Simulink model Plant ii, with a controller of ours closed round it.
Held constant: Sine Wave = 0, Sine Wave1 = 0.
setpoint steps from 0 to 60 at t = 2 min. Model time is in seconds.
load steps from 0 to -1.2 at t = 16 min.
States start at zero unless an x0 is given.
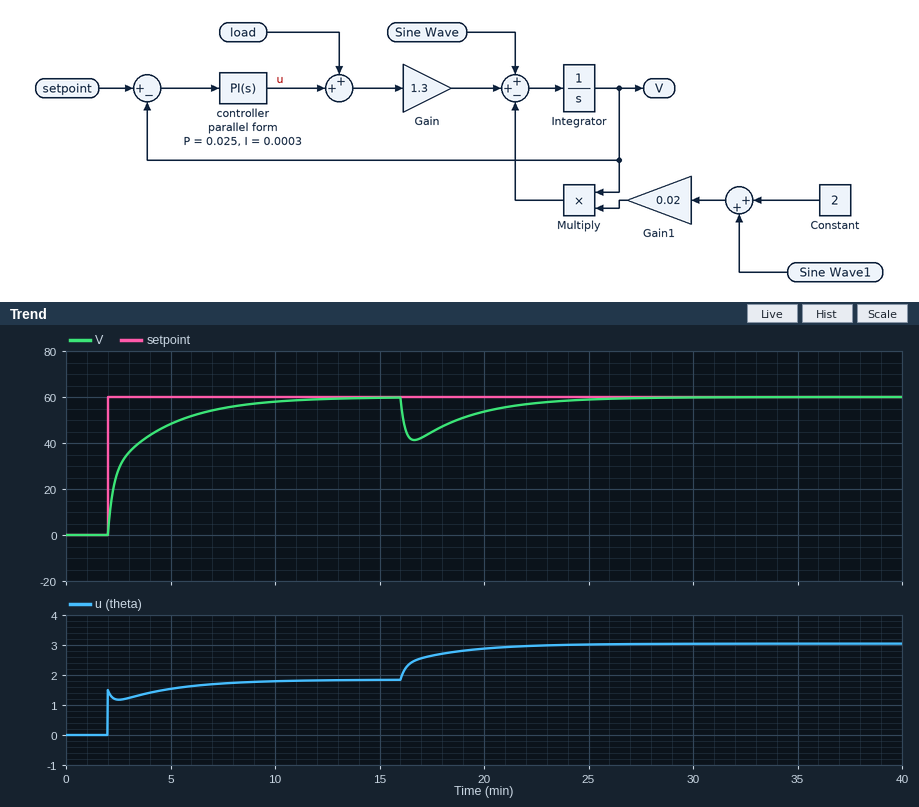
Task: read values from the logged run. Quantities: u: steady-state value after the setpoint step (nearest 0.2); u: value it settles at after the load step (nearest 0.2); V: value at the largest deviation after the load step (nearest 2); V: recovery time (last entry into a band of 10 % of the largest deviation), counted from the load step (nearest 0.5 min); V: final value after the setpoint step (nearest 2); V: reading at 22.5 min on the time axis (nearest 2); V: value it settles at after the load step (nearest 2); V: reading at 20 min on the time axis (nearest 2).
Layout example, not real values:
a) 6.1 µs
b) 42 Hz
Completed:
a) 1.8
b) 3.0
c) 42
d) 7.5 min
e) 60
f) 58
g) 60
h) 54
